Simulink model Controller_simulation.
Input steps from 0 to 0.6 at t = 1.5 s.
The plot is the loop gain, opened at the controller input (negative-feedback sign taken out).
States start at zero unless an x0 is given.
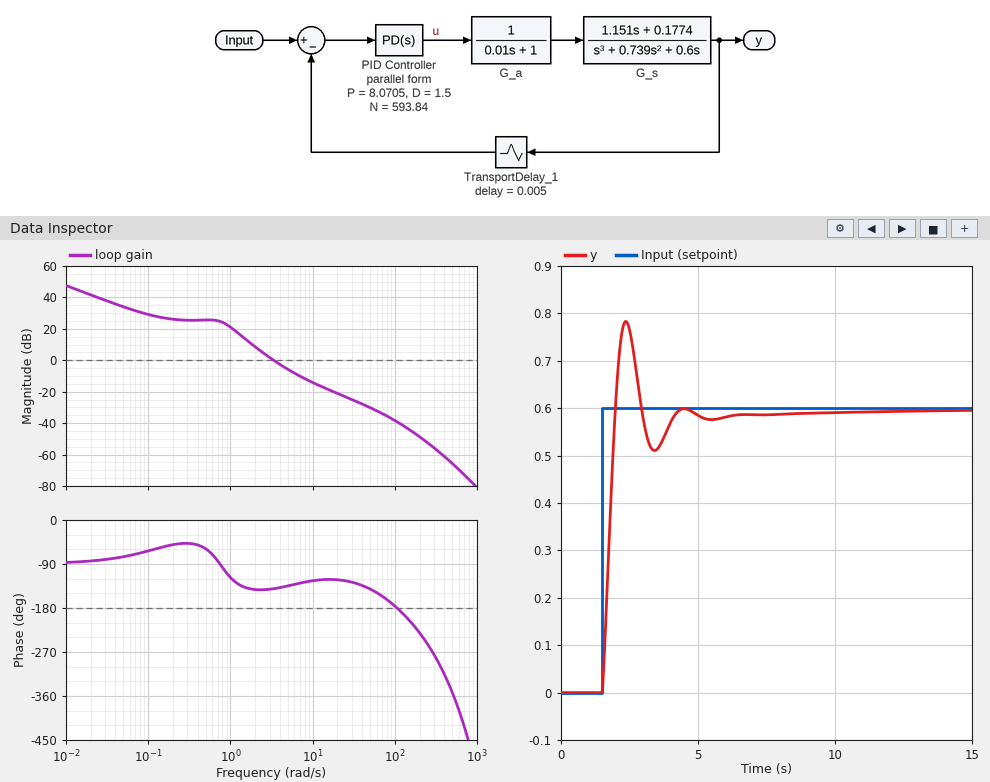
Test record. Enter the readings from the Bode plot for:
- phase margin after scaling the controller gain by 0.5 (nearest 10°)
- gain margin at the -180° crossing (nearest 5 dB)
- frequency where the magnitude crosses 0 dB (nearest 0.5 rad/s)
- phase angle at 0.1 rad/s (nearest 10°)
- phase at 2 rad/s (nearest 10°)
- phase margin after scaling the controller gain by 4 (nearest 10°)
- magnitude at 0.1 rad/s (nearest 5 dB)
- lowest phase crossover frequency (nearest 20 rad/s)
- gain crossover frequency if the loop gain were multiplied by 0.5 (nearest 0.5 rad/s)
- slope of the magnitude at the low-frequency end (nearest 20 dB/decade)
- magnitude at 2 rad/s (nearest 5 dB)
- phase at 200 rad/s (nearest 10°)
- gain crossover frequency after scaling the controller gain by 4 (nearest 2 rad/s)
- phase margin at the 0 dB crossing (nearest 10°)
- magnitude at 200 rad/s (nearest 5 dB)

40°
40 dB
3.5 rad/s
-60°
-140°
50°
30 dB
100 rad/s
2.5 rad/s
-20 dB/decade
10 dB
-230°
8 rad/s
40°
-50 dB
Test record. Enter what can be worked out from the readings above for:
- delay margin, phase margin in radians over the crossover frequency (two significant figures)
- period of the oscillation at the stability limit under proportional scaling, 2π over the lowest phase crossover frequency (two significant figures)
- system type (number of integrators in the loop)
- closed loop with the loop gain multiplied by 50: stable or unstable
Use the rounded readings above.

0.20 s
0.063 s
1
stable
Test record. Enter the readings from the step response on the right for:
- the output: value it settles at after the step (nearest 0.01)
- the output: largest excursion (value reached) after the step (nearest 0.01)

0.60
0.78
